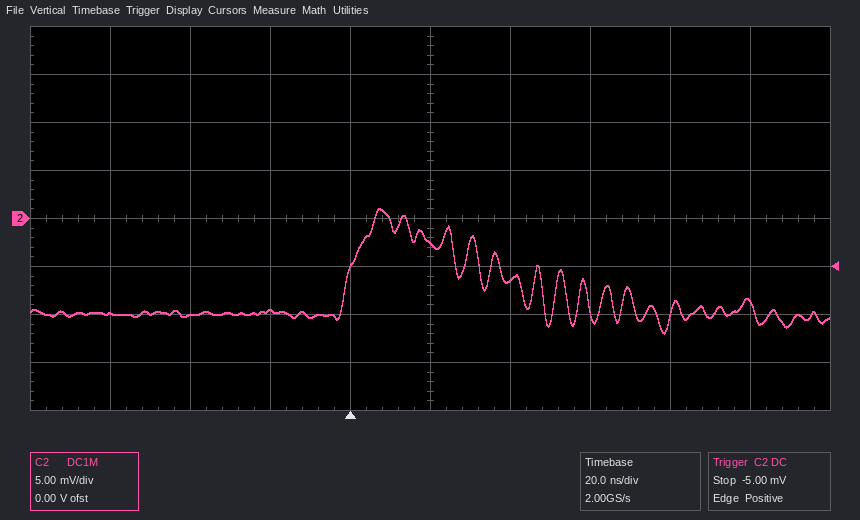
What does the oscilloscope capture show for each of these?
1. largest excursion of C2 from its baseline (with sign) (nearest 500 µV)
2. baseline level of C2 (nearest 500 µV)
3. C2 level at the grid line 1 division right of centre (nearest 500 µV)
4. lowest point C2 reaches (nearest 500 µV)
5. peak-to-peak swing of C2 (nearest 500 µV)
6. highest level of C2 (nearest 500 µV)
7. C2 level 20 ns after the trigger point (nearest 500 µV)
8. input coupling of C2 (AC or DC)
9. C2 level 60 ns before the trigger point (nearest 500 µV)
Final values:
+11.0 mV
-10.0 mV
-6.5 mV
-12.0 mV
13.0 mV
1.0 mV
-2.5 mV
DC
-10.0 mV
